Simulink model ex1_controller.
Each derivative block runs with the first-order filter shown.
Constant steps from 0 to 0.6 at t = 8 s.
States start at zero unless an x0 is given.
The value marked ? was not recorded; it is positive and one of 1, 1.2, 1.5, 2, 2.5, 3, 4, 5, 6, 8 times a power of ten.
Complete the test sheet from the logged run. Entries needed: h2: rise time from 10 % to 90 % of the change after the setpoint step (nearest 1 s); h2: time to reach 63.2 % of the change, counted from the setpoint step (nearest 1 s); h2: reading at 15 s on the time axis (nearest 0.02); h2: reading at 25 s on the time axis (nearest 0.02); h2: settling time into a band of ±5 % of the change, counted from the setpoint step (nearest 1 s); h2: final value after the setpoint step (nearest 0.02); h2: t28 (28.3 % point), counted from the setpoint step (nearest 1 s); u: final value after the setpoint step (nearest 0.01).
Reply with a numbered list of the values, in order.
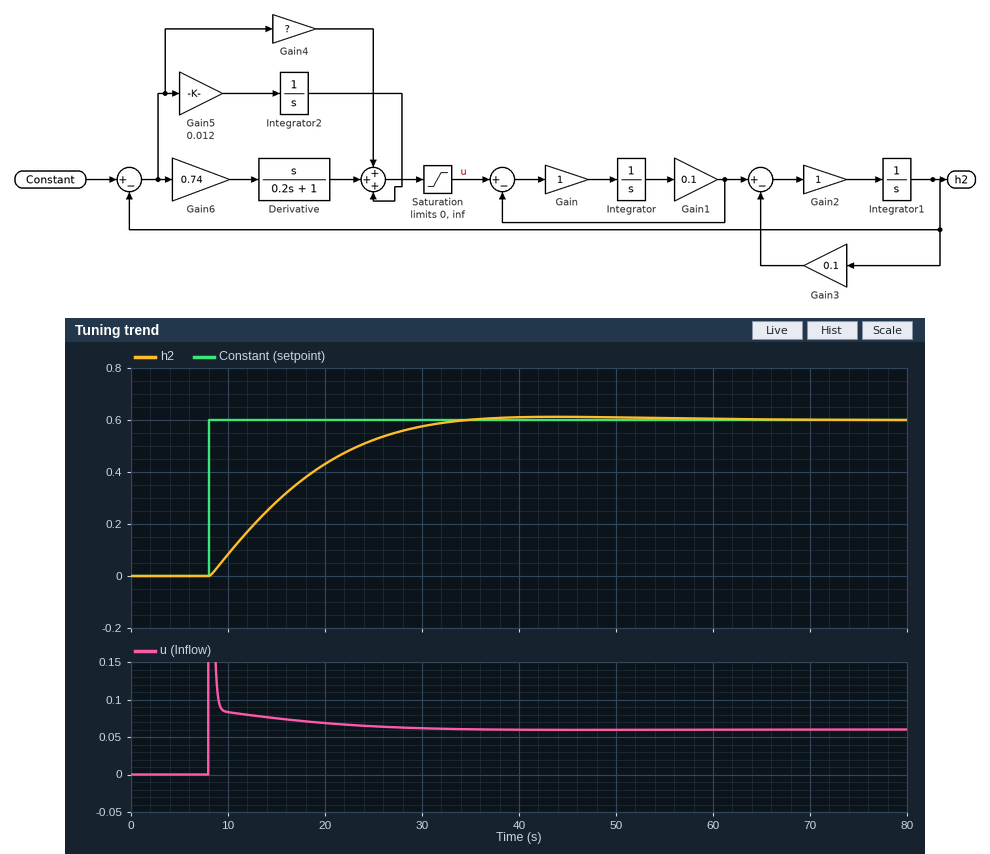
1. 17 s
2. 10 s
3. 0.28
4. 0.52
5. 21 s
6. 0.60
7. 4 s
8. 0.06
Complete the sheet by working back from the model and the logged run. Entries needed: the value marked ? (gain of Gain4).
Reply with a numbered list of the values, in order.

1. 0.2
